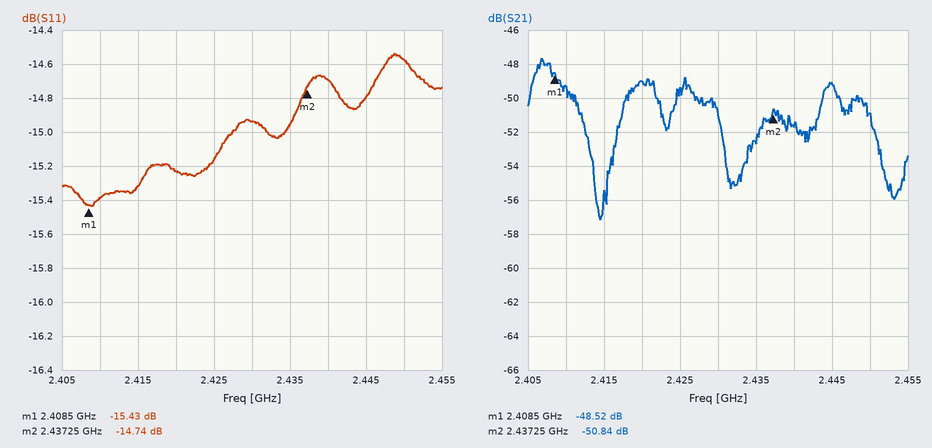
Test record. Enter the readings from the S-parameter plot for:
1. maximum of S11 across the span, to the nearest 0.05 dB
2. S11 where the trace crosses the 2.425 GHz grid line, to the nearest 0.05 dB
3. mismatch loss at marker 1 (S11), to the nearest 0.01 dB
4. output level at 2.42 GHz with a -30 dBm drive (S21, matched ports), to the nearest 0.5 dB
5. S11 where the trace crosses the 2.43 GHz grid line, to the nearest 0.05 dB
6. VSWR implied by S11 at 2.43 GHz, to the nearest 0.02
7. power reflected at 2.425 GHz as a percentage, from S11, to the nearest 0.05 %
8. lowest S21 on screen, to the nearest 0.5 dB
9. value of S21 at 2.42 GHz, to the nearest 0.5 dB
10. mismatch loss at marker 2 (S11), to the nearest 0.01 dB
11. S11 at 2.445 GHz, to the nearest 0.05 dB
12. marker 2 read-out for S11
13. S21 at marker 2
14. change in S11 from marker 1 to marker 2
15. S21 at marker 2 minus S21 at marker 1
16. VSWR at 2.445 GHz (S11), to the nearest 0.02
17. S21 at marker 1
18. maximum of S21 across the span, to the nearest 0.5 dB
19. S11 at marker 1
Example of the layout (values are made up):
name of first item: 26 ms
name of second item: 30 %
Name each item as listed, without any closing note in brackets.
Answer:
maximum of S11 across the span, to the nearest 0.05 dB: -14.55 dB
S11 where the trace crosses the 2.425 GHz grid line, to the nearest 0.05 dB: -15.15 dB
mismatch loss at marker 1 (S11), to the nearest 0.01 dB: 0.13 dB
output level at 2.42 GHz with a -30 dBm drive (S21, matched ports), to the nearest 0.5 dB: -79.0 dBm
S11 where the trace crosses the 2.43 GHz grid line, to the nearest 0.05 dB: -14.95 dB
VSWR implied by S11 at 2.43 GHz, to the nearest 0.02: 1.44
power reflected at 2.425 GHz as a percentage, from S11, to the nearest 0.05 %: 3.05 %
lowest S21 on screen, to the nearest 0.5 dB: -57.0 dB
value of S21 at 2.42 GHz, to the nearest 0.5 dB: -49.0 dB
mismatch loss at marker 2 (S11), to the nearest 0.01 dB: 0.15 dB
S11 at 2.445 GHz, to the nearest 0.05 dB: -14.80 dB
marker 2 read-out for S11: -14.74 dB
S21 at marker 2: -50.84 dB
change in S11 from marker 1 to marker 2: 0.69 dB
S21 at marker 2 minus S21 at marker 1: -2.32 dB
VSWR at 2.445 GHz (S11), to the nearest 0.02: 1.44
S21 at marker 1: -48.52 dB
maximum of S21 across the span, to the nearest 0.5 dB: -47.5 dB
S11 at marker 1: -15.43 dB
